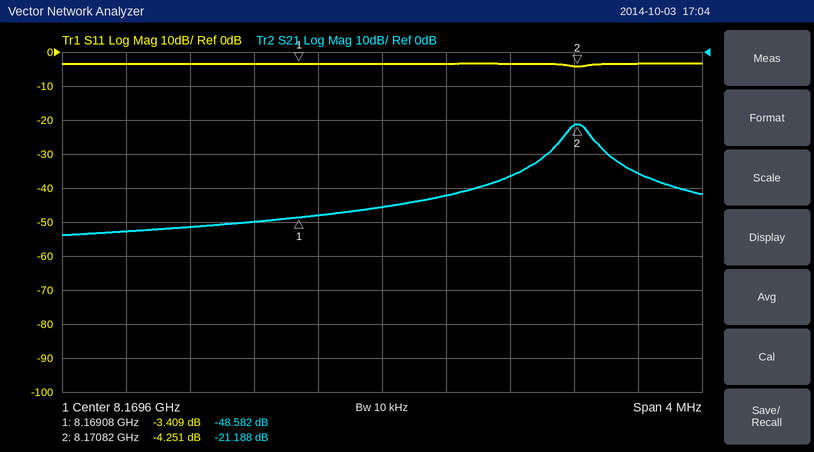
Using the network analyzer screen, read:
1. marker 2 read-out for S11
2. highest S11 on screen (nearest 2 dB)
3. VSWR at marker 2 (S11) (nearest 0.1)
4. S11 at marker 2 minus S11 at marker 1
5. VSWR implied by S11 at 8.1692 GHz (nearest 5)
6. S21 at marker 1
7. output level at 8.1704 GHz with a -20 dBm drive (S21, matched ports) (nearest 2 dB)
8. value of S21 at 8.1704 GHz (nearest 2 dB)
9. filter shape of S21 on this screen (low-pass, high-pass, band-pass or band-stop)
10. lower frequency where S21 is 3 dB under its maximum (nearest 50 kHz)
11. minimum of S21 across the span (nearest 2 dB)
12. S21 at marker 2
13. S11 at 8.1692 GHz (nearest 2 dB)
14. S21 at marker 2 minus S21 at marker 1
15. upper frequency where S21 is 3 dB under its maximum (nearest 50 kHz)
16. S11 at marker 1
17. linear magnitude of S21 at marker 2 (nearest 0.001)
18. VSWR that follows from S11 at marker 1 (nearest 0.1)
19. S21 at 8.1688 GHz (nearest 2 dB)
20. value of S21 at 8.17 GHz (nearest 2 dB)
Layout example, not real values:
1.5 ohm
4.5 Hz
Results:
-4.251 dB
-4 dB
4.2
-0.842 dB
5
-48.582 dB
-56 dBm
-36 dB
band-pass
8.17075 GHz
-54 dB
-21.188 dB
-4 dB
27.394 dB
8.17090 GHz
-3.409 dB
0.087
5.2
-50 dB
-42 dB
